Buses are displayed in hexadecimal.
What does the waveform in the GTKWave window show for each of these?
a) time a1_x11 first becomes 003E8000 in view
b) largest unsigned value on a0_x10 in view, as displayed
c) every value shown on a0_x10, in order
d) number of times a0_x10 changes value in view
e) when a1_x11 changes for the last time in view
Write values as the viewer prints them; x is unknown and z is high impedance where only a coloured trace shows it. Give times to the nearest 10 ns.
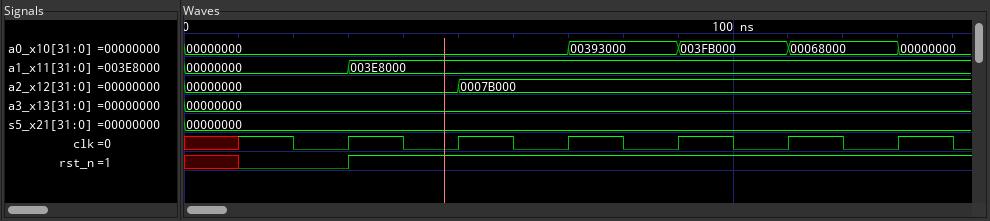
30 ns
003FB000
00000000, 00393000, 003FB000, 00068000, 00000000
4
30 ns
